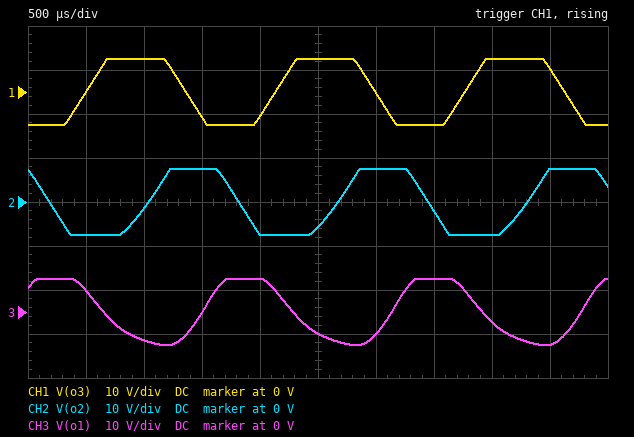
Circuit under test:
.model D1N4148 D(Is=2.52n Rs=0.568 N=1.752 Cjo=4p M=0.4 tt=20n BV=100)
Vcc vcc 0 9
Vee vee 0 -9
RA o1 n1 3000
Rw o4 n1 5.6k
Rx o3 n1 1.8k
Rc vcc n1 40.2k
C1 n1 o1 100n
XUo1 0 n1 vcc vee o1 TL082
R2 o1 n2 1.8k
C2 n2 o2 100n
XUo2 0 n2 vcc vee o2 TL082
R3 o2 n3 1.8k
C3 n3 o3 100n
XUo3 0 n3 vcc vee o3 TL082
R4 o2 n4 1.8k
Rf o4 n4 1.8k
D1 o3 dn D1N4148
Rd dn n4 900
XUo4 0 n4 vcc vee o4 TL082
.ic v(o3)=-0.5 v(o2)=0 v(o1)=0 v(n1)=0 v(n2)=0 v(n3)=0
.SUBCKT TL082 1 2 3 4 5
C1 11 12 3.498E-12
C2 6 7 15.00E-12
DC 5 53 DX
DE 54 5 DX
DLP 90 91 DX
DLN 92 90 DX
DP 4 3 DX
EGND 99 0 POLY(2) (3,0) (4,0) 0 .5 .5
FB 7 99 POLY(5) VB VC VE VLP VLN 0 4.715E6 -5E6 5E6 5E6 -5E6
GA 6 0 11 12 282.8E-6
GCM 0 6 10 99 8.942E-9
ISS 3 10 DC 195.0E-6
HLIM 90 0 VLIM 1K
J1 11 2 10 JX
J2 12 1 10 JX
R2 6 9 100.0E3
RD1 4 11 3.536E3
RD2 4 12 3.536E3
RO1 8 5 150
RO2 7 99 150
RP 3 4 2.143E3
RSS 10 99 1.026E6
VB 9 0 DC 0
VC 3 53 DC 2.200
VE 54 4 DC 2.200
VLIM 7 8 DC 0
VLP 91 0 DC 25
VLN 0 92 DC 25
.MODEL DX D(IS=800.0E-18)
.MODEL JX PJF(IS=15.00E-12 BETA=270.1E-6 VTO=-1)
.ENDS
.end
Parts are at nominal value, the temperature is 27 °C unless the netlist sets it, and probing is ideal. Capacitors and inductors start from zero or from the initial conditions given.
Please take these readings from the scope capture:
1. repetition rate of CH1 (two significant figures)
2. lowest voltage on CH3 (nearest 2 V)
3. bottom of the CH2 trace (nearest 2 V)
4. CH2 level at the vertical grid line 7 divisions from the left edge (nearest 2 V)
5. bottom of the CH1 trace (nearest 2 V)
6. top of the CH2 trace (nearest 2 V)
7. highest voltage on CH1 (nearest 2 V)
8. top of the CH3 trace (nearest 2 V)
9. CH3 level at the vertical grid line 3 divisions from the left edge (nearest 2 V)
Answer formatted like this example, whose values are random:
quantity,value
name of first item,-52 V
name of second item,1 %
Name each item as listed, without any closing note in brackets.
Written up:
quantity,value
repetition rate of CH1,610 Hz
lowest voltage on CH3,-8 V
bottom of the CH2 trace,-8 V
CH2 level at the vertical grid line 7 divisions from the left edge,-2 V
bottom of the CH1 trace,-8 V
top of the CH2 trace,8 V
highest voltage on CH1,8 V
top of the CH3 trace,8 V
CH3 level at the vertical grid line 3 divisions from the left edge,0 V
